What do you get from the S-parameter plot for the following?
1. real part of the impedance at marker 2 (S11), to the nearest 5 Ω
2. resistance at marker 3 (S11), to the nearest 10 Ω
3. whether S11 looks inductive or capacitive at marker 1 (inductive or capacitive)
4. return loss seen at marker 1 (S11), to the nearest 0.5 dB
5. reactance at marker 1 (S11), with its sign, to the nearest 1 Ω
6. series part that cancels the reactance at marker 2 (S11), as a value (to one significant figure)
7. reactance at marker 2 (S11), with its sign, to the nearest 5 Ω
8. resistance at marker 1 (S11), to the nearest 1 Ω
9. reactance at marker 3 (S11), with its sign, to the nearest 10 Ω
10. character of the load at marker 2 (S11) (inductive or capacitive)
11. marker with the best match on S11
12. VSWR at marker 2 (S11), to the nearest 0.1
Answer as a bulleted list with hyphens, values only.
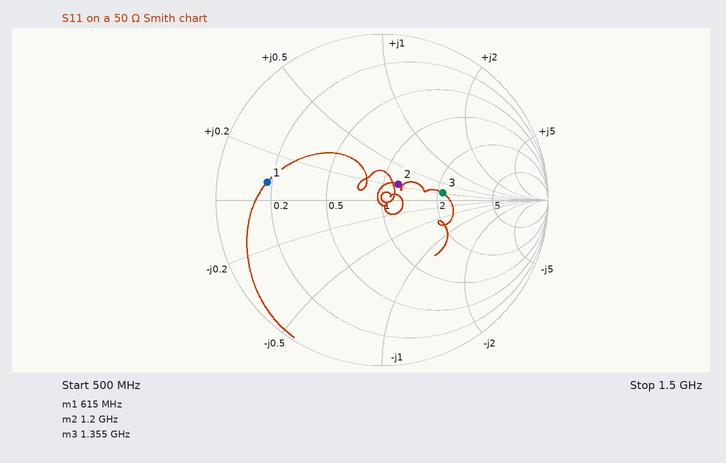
- 60 Ω
- 110 Ω
- inductive
- 3.0 dB
- +4 Ω
- 10 pF
- +10 Ω
- 9 Ω
- +10 Ω
- inductive
- marker 2
- 1.3
